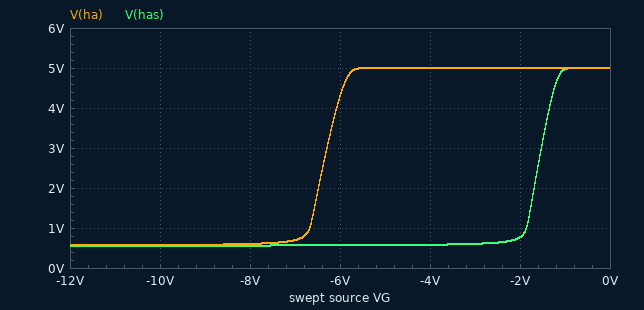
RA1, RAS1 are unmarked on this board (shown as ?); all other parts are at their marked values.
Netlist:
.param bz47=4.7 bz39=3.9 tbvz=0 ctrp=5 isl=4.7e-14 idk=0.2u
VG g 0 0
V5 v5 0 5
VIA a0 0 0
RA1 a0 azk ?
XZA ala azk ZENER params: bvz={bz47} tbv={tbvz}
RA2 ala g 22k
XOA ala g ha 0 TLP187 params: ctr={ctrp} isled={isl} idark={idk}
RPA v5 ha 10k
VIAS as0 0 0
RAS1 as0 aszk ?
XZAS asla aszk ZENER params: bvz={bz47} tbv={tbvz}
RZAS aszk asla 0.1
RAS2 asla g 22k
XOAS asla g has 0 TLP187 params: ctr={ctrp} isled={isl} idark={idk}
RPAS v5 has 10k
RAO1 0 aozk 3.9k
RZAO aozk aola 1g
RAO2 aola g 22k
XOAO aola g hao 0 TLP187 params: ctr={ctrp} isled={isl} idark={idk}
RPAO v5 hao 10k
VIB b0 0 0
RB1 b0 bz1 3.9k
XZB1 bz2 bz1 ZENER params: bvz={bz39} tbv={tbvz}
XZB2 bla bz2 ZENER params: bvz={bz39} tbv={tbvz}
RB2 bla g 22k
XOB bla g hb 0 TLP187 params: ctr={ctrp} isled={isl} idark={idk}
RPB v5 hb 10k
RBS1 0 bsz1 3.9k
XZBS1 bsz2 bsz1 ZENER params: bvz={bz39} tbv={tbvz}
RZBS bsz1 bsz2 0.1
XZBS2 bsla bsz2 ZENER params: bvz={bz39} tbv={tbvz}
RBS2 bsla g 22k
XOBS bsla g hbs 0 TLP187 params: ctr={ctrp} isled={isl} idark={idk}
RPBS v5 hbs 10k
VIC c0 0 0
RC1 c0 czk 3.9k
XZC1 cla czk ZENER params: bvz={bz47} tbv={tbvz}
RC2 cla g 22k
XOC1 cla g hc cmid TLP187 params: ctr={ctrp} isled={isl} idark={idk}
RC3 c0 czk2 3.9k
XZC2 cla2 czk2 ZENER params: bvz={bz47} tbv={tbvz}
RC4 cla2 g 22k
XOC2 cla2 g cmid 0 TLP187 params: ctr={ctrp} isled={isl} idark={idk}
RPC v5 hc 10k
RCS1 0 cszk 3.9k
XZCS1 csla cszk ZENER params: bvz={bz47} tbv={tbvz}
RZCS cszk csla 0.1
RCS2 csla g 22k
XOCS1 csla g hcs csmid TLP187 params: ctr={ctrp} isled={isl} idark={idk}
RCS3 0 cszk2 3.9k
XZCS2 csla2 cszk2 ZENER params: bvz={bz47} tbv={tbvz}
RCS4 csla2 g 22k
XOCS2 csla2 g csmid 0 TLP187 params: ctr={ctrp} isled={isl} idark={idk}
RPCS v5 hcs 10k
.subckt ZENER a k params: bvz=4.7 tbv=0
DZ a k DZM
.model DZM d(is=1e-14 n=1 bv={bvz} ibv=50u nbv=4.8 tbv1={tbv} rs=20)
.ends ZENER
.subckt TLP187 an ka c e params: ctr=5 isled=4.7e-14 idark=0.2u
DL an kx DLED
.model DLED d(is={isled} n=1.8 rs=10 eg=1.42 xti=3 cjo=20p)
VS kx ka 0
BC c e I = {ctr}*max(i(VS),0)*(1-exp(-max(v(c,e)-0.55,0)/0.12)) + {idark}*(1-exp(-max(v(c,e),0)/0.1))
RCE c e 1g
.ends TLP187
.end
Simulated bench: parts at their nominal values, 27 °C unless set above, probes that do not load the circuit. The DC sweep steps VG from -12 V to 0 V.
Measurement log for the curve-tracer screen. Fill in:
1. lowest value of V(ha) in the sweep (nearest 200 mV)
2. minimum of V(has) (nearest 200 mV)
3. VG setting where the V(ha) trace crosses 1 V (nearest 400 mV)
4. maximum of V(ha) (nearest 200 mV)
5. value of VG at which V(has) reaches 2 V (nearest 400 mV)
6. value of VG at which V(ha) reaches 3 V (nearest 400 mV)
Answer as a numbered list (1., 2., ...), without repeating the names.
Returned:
1. 600 mV
2. 600 mV
3. -6.8 V
4. 5.0 V
5. -1.6 V
6. -6.4 V
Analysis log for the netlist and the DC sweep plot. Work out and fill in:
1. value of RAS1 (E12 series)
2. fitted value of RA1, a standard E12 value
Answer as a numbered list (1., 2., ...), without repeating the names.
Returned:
1. 6.8 kΩ
2. 6.8 kΩ
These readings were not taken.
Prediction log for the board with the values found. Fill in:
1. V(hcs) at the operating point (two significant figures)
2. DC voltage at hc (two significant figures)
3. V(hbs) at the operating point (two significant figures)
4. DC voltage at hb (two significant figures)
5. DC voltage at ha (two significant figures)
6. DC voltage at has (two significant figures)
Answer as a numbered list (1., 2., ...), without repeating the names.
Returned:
1. 5.0 V
2. 5.0 V
3. 5.0 V
4. 5.0 V
5. 5.0 V
6. 5.0 V
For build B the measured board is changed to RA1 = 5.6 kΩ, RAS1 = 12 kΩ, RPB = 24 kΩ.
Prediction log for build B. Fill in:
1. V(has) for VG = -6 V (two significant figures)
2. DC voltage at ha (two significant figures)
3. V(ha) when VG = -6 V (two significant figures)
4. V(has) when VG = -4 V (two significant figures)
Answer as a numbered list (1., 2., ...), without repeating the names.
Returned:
1. 580 mV
2. 5.0 V
3. 4.0 V
4. 620 mV
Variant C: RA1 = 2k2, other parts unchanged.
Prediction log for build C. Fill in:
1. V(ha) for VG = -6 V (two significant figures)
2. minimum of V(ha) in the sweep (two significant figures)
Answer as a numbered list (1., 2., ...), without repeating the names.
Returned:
1. 2.0 V
2. 550 mV
